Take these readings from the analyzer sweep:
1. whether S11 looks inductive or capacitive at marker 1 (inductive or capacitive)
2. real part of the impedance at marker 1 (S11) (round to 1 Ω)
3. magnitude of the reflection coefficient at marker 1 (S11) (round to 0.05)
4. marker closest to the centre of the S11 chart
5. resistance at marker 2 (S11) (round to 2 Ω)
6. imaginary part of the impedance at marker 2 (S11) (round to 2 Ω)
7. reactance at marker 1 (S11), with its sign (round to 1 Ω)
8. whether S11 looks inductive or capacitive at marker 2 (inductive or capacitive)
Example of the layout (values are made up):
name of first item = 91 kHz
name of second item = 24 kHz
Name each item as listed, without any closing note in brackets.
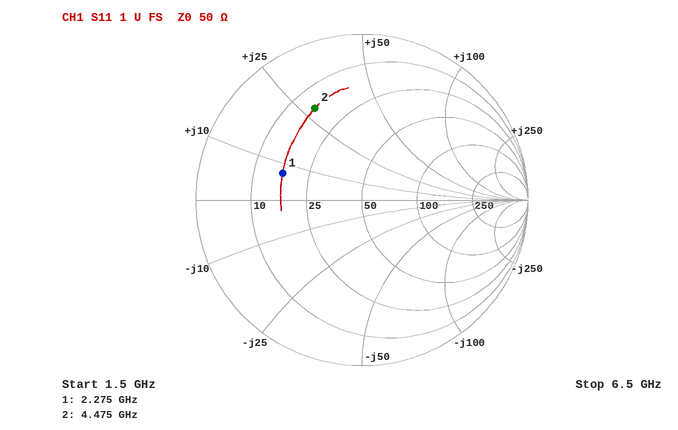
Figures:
whether S11 looks inductive or capacitive at marker 1 = inductive
real part of the impedance at marker 1 (S11) = 17 Ω
magnitude of the reflection coefficient at marker 1 (S11) = 0.50
marker closest to the centre of the S11 chart = marker 1
resistance at marker 2 (S11) = 16 Ω
imaginary part of the impedance at marker 2 (S11) = +28 Ω
reactance at marker 1 (S11), with its sign = +7 Ω
whether S11 looks inductive or capacitive at marker 2 = inductive
